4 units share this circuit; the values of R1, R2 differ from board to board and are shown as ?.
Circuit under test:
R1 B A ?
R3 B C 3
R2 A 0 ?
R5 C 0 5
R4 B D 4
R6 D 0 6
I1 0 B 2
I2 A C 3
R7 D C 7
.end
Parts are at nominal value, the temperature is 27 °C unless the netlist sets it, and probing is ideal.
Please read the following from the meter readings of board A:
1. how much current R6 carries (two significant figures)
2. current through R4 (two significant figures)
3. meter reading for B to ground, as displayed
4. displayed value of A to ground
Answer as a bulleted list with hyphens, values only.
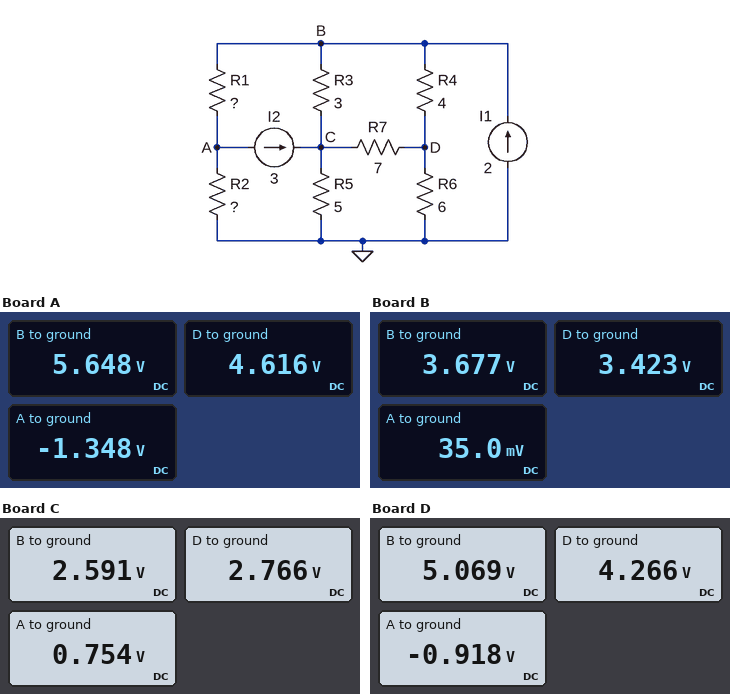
- 770 mA
- 260 mA
- 5.648 V
- -1.348 V
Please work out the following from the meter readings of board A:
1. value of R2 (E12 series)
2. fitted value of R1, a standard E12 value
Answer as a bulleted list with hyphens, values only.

- 3.3 Ω
- 2.7 Ω
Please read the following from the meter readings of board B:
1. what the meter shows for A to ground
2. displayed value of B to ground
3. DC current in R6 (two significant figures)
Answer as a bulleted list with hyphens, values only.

- 35.0 mV
- 3.677 V
- 570 mA
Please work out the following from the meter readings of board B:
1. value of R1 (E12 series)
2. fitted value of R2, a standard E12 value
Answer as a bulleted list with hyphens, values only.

- 1.2 Ω
- 1 Ω
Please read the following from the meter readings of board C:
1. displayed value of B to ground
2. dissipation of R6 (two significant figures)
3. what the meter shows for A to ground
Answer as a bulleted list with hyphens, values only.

- 2.591 V
- 1.3 W
- 0.754 V
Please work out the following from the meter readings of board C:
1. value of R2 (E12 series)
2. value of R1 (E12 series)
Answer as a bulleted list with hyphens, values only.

- 2.7 Ω
- 0.56 Ω
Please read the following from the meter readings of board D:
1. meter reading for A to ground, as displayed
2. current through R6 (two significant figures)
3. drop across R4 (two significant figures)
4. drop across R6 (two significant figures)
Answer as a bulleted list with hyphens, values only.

- -0.918 V
- 710 mA
- 800 mV
- 4.3 V
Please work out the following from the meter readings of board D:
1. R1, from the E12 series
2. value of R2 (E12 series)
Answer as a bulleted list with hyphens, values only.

- 2.2 Ω
- 3.3 Ω
